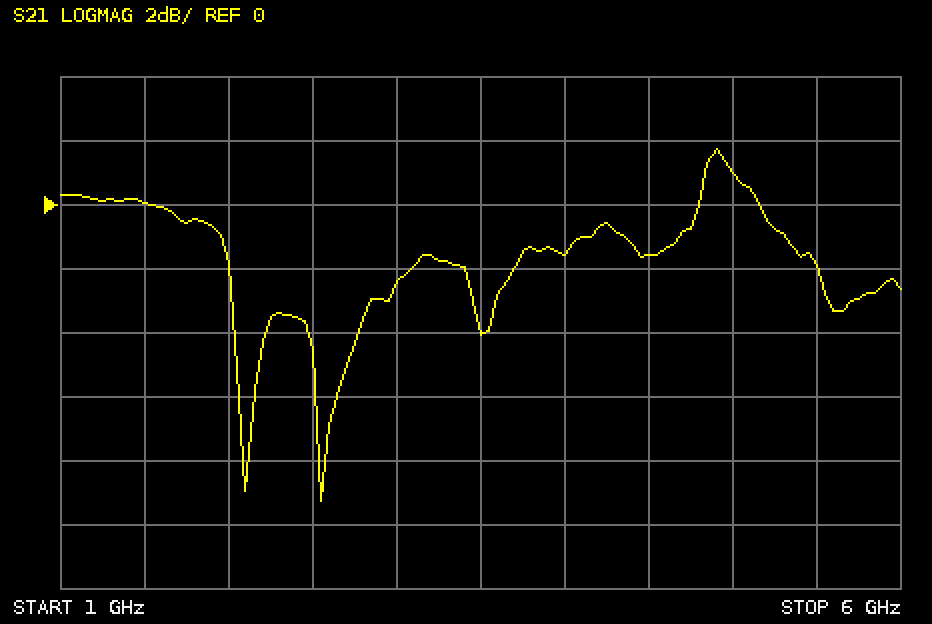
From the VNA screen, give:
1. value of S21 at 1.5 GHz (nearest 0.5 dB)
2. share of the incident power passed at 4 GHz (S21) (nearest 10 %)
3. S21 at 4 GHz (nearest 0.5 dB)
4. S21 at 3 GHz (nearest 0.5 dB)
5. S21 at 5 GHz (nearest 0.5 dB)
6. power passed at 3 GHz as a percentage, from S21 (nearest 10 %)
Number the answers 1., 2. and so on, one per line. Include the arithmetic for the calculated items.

1. 0.0 dB
2. 10^(-1.5/10) ≈ 70.8 %, so 70 % to the nearest 10 %
3. -1.5 dB
4. -2.5 dB
5. 1.0 dB
6. 10^(-2.5/10) ≈ 56.2 %, so 60 % to the nearest 10 %
